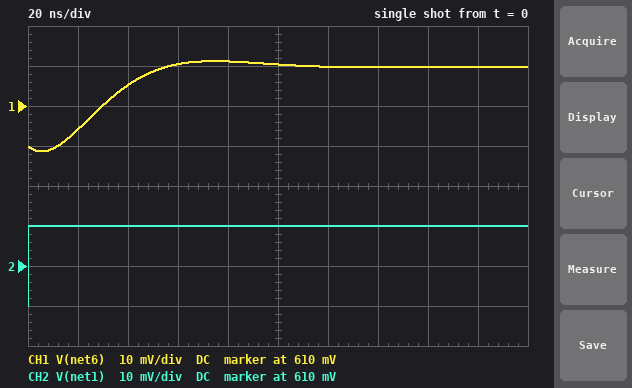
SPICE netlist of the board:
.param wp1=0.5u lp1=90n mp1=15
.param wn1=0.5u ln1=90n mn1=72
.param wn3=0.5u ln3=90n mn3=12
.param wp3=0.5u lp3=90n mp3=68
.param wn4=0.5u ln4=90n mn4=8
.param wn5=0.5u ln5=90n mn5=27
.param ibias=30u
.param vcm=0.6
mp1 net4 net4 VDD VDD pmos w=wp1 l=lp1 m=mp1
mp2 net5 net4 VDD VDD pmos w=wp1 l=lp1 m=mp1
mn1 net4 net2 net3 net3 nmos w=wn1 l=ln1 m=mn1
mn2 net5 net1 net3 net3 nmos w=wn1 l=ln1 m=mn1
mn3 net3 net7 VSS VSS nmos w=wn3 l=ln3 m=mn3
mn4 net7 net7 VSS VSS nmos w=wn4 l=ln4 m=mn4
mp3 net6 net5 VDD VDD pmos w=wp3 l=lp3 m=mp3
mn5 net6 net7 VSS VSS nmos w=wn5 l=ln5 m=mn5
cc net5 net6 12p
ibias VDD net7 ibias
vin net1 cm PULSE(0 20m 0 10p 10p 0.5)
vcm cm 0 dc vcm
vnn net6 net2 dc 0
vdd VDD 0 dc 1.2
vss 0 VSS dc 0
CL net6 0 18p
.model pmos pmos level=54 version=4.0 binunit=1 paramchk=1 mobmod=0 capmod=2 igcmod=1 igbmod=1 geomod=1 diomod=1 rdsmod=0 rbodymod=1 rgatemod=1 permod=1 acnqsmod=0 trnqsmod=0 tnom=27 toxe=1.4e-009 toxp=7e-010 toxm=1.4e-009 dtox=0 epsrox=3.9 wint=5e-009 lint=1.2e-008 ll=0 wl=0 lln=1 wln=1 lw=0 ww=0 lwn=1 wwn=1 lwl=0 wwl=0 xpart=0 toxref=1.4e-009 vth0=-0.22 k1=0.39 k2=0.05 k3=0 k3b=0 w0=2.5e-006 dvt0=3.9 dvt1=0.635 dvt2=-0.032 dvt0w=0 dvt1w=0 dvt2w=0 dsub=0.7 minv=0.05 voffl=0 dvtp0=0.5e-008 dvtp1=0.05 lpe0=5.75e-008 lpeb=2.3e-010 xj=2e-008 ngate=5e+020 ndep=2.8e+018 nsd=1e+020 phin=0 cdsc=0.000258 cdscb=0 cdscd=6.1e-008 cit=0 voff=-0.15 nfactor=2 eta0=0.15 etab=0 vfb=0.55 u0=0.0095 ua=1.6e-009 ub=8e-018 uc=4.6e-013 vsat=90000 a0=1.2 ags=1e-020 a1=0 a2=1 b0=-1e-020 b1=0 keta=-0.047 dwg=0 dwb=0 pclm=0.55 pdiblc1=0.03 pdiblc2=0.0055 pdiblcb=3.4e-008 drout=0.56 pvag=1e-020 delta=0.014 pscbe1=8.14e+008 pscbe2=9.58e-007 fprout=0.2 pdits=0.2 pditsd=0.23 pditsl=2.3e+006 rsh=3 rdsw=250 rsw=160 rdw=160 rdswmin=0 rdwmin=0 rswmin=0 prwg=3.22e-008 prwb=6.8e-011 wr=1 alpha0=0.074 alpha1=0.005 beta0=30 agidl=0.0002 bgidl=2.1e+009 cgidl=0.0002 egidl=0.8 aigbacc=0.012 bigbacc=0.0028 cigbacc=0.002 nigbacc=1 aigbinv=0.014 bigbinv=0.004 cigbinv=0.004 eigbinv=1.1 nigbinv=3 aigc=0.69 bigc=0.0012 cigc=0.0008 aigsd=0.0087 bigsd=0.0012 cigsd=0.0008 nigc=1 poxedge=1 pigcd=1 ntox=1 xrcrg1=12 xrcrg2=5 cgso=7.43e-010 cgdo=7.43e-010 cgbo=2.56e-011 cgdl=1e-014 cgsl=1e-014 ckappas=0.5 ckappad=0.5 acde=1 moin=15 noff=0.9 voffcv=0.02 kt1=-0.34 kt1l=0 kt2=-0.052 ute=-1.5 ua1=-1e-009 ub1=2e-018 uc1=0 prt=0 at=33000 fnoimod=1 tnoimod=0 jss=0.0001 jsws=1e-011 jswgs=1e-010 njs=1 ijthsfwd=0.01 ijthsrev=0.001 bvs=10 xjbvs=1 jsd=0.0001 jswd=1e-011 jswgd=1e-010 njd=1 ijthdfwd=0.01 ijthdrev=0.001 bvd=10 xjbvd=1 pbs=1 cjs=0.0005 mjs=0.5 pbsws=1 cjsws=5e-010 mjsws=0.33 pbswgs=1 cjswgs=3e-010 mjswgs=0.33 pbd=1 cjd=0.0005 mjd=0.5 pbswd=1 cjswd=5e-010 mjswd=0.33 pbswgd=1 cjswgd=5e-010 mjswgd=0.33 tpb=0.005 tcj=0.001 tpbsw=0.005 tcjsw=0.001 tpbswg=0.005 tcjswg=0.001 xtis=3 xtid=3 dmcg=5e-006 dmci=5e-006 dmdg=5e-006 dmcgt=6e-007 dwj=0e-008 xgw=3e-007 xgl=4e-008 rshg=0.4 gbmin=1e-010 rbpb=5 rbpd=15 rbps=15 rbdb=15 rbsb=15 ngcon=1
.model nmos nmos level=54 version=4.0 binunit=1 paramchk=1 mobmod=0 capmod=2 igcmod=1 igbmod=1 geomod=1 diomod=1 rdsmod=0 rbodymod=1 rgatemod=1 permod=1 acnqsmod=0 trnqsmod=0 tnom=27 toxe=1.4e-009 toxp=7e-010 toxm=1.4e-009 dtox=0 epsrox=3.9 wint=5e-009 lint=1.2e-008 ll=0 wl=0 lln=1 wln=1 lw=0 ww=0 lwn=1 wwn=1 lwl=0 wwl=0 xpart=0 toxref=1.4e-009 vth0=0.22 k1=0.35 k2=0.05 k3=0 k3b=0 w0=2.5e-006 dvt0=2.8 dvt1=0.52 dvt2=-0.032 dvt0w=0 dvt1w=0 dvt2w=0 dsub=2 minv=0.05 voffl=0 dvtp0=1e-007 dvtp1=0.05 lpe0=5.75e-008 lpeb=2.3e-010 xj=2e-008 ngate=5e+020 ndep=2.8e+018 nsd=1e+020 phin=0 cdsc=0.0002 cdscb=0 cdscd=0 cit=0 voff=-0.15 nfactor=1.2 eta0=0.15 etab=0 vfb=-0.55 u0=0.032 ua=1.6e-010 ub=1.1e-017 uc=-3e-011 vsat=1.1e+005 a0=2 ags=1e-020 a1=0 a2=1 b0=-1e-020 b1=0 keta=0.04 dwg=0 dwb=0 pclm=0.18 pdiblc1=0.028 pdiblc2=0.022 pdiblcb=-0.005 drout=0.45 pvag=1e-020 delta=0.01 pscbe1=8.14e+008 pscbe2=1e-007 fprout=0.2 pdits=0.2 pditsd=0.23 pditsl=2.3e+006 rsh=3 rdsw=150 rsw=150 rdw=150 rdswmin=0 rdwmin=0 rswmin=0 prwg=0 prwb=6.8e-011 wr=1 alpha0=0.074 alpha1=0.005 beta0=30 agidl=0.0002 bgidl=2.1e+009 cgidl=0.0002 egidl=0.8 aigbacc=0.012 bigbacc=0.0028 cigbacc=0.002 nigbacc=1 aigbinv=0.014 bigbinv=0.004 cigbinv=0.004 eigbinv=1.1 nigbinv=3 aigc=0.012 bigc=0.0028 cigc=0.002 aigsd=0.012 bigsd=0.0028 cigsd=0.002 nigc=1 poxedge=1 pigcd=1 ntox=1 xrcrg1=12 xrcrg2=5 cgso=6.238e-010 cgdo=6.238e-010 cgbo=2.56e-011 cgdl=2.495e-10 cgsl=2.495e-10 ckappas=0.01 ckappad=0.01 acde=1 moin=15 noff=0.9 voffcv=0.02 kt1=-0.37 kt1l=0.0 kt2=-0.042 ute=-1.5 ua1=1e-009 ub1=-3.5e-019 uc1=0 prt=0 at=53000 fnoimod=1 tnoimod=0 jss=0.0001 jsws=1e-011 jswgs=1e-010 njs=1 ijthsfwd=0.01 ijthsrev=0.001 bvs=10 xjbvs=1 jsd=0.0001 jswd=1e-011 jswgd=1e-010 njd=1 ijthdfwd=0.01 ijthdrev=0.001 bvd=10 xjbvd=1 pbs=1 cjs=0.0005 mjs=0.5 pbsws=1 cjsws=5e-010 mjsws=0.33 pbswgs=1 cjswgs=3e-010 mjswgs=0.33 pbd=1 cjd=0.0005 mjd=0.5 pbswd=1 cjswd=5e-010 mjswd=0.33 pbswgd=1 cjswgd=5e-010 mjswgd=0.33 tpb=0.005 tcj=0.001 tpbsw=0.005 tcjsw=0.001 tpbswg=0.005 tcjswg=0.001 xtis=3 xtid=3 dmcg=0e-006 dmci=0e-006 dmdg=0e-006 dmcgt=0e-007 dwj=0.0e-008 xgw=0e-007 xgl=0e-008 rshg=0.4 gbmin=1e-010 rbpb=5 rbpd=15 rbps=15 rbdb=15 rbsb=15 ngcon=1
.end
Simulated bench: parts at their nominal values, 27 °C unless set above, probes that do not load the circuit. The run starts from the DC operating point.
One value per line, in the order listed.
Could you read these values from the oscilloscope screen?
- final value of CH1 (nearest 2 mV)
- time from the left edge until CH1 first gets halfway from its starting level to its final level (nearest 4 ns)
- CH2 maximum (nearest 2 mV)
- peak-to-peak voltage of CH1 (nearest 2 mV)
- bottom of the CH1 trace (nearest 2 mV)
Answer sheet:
620 mV
28 ns
620 mV
22 mV
598 mV
